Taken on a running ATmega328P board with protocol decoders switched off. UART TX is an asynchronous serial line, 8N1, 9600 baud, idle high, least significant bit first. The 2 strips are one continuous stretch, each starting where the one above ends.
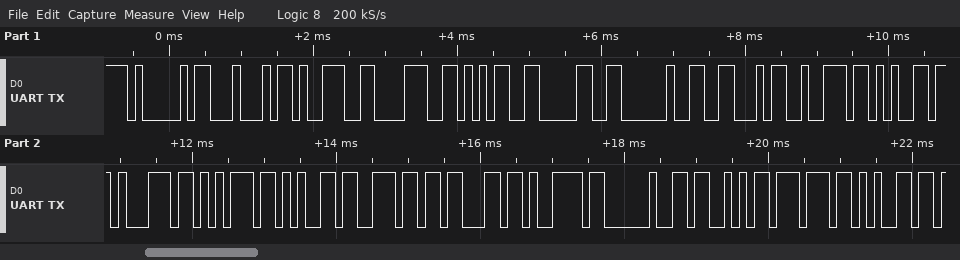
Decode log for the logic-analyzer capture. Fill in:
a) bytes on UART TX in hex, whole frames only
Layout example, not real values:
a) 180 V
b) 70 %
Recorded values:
a) 41 44 39 38 35 30 20 46 72 65 71 75 65 6E 63 79 20 53 77 65
